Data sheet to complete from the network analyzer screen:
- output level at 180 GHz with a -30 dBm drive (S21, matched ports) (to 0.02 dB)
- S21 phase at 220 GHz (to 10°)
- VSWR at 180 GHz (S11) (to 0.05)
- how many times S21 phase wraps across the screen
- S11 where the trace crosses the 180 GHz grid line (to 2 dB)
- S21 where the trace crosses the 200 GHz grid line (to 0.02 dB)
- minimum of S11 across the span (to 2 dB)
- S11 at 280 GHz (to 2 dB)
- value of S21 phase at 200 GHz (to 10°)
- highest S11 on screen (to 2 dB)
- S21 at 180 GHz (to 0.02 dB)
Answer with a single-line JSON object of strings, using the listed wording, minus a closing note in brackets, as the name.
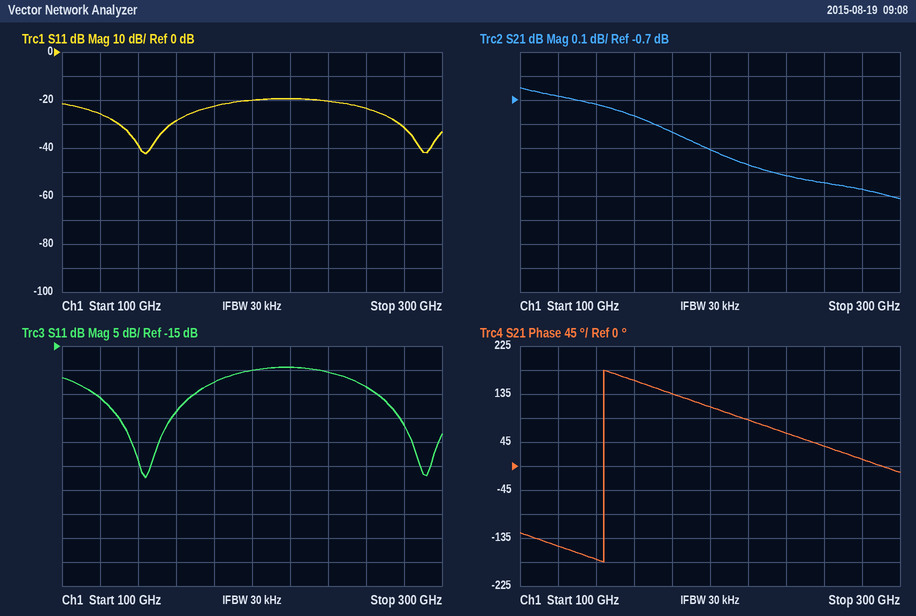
{"output level at 180 GHz with a -30 dBm drive (S21, matched ports)": "-30.84 dBm", "S21 phase at 220 GHz": "90°", "VSWR at 180 GHz (S11)": "1.15", "how many times S21 phase wraps across the screen": "1", "S11 where the trace crosses the 180 GHz grid line": "-22 dB", "S21 where the trace crosses the 200 GHz grid line": "-0.90 dB", "minimum of S11 across the span": "-42 dB", "S11 at 280 GHz": "-32 dB", "value of S21 phase at 200 GHz": "110°", "highest S11 on screen": "-20 dB", "S21 at 180 GHz": "-0.84 dB"}
